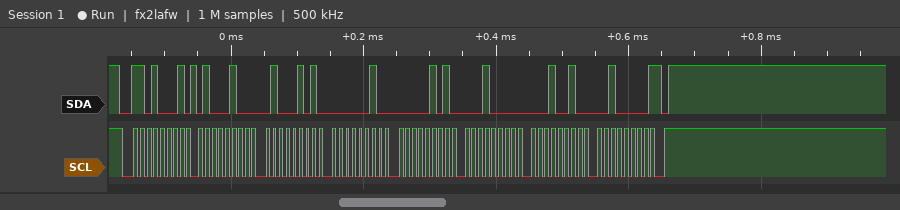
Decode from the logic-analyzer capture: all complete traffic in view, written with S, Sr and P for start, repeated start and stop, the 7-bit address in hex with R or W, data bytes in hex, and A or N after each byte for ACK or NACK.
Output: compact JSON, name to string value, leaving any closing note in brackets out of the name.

{"all complete traffic in view, written with S, Sr and P for start, repeated start and stop, the 7-bit address in hex with R or W, data bytes in hex, and A or N after each byte for ACK or NACK": "S 68R A 44 A 45 A 02 A 05 A 10 A 12 A 20 N P"}
